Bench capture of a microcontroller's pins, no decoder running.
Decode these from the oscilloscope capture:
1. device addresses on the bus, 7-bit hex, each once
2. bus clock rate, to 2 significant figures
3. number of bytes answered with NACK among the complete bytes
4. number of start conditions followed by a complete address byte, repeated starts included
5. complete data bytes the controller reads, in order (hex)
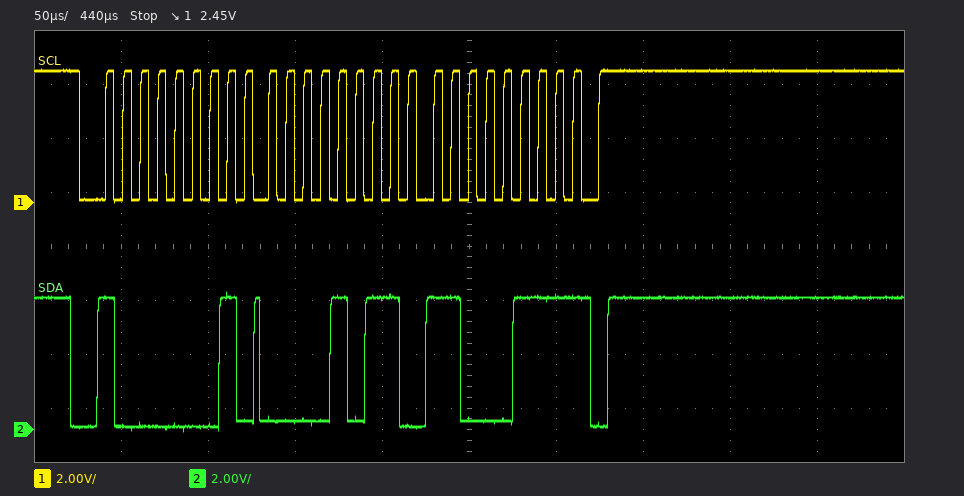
0x40
100 kHz
1
1
0B C7
